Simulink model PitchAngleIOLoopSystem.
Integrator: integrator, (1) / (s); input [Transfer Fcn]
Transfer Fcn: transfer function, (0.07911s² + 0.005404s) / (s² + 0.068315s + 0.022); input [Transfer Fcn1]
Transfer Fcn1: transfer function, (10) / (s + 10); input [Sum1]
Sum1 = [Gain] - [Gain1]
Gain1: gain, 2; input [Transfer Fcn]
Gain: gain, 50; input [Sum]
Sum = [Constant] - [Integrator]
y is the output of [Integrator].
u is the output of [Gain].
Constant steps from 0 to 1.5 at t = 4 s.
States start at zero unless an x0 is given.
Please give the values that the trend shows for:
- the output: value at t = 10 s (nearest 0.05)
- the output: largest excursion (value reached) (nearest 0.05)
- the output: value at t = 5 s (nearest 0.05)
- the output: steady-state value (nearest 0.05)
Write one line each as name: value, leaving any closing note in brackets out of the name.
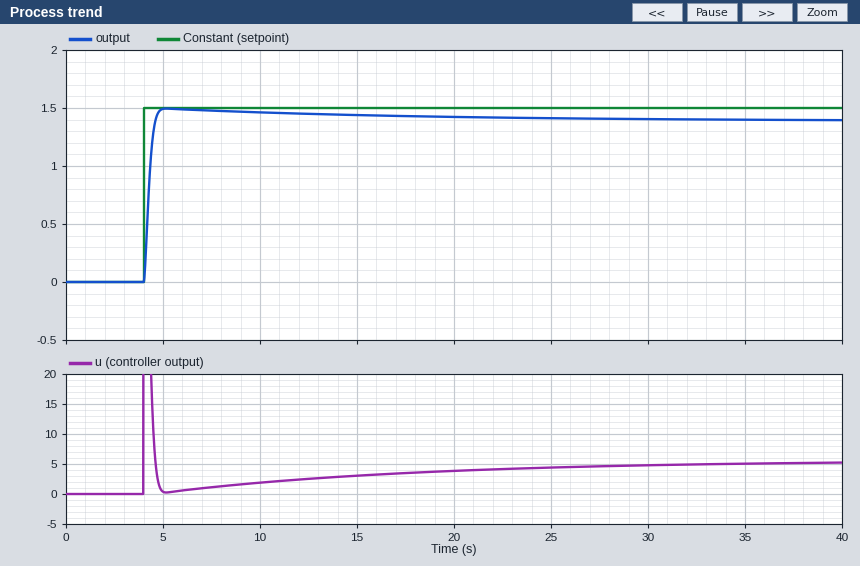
the output: value at t = 10 s: 1.45
the output: largest excursion (value reached): 1.50
the output: value at t = 5 s: 1.50
the output: steady-state value: 1.40
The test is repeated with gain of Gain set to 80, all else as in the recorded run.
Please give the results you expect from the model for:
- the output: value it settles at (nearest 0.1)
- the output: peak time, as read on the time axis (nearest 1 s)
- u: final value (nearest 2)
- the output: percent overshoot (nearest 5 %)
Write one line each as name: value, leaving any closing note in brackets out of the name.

the output: value it settles at: 1.4
the output: peak time, as read on the time axis: 5 s
u: final value: 6
the output: percent overshoot: 10 %
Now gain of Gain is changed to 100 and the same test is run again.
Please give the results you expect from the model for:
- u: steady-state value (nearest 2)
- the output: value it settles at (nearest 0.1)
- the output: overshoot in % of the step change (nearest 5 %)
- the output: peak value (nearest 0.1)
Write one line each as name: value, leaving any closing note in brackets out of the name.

u: steady-state value: 6
the output: value it settles at: 1.4
the output: overshoot in % of the step change: 10 %
the output: peak value: 1.6
